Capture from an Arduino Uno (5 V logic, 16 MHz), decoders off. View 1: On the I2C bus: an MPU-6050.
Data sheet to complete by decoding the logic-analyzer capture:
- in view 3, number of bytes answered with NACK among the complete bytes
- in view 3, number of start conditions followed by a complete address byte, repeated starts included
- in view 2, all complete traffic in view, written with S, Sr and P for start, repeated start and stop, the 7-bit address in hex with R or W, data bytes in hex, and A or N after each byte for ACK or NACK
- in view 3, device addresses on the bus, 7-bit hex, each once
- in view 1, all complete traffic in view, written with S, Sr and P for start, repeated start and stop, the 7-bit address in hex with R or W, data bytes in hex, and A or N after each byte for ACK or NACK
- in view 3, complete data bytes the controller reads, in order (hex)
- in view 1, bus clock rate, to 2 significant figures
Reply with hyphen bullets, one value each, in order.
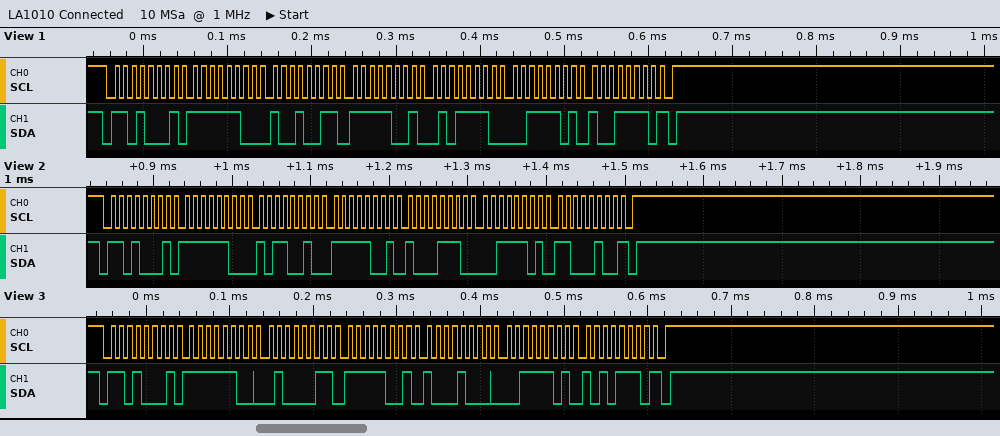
- 1
- 1
- S 68R A FC A B2 A F9 A 8E A 3D A C4 N P
- 0x68
- S 68R A FC A 93 A F9 A 5E A 3D A 9E N P
- FC 43 F9 88 3D AE
- 100 kHz
